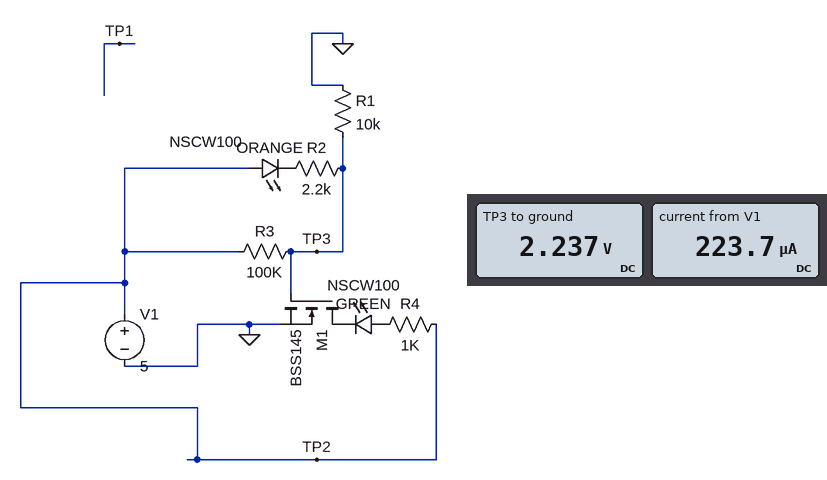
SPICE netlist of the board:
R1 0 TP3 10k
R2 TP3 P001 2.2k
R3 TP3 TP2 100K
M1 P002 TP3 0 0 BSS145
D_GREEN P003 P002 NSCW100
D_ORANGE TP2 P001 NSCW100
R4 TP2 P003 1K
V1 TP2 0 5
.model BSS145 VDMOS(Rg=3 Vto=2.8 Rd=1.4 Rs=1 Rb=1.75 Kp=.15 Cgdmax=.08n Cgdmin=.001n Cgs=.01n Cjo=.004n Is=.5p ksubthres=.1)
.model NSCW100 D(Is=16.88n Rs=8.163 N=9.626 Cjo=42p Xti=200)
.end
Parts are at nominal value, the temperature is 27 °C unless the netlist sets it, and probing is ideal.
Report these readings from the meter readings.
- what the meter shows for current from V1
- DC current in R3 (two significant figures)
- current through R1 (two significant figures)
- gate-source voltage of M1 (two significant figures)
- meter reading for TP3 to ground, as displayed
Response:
223.7 µA
28 µA
220 µA
2.2 V
2.237 V
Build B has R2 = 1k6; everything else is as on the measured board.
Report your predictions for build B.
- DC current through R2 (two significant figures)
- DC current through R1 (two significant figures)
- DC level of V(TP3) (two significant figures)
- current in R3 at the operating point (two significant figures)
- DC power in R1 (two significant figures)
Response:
210 µA
230 µA
2.3 V
27 µA
540 µW
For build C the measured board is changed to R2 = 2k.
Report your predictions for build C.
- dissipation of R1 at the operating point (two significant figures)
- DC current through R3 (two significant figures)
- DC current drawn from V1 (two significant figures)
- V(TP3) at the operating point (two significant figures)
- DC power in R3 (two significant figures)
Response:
510 µW
27 µA
230 µA
2.3 V
75 µW
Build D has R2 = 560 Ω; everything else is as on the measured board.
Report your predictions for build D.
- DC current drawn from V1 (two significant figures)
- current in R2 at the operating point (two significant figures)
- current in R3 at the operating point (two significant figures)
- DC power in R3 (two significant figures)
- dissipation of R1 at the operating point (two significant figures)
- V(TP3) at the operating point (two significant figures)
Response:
250 µA
230 µA
25 µA
62 µW
630 µW
2.5 V
